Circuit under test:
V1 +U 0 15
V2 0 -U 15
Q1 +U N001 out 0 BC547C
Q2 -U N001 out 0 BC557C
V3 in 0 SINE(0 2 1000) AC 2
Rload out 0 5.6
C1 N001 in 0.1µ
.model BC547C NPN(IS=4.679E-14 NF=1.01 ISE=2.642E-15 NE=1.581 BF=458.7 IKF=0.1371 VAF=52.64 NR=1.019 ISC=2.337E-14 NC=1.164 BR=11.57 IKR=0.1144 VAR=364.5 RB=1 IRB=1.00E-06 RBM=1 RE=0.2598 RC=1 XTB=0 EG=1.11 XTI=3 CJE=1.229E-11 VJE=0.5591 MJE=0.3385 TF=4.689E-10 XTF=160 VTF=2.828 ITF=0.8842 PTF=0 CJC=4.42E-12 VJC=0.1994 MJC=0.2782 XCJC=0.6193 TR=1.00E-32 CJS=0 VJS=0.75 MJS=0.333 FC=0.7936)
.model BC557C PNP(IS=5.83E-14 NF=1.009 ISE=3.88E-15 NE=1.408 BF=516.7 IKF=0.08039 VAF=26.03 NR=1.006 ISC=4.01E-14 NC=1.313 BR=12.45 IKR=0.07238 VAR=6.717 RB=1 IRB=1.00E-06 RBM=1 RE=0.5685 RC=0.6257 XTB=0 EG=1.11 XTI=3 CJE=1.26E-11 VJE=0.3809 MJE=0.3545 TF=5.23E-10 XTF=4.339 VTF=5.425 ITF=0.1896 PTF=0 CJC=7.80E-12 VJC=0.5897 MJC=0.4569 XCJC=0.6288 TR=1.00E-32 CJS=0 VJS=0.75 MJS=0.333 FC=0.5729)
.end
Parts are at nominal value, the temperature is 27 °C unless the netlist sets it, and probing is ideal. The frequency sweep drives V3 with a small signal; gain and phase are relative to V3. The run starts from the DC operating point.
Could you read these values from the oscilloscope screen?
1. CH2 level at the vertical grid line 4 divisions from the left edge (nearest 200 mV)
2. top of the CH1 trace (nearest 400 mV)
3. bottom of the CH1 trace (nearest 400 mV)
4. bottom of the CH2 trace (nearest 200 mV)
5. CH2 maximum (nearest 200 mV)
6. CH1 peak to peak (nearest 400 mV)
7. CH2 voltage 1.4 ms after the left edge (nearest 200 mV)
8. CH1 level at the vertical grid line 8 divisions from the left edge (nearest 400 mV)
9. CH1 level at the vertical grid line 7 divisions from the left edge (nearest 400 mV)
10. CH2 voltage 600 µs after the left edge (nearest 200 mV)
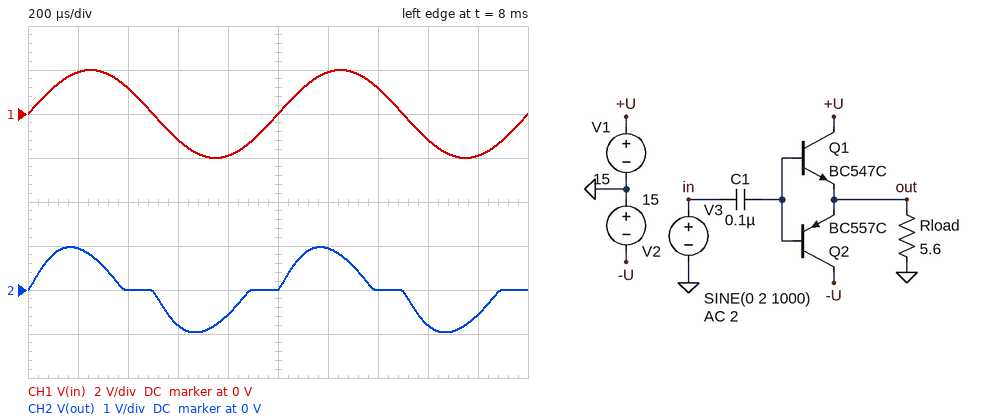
-600 mV
2.0 V
-2.0 V
-1.0 V
1.0 V
4.0 V
0 V
-1.2 V
1.2 V
-800 mV
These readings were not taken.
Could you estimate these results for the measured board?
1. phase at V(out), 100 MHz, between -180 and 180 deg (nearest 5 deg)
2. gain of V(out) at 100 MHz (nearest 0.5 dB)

85 deg
-21.0 dB
